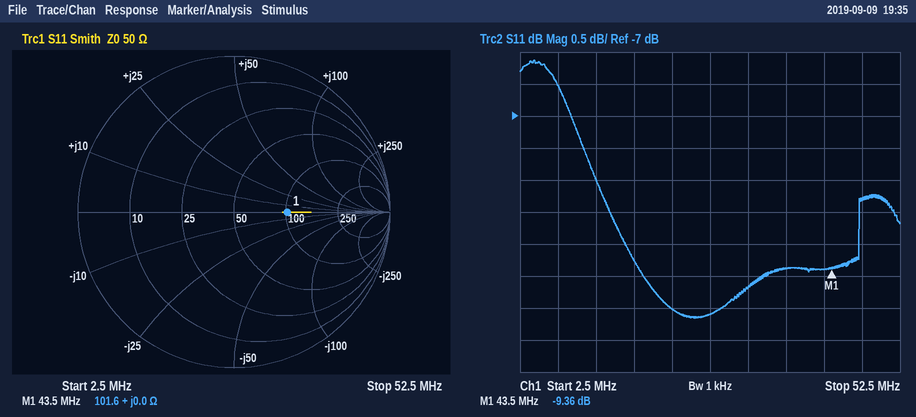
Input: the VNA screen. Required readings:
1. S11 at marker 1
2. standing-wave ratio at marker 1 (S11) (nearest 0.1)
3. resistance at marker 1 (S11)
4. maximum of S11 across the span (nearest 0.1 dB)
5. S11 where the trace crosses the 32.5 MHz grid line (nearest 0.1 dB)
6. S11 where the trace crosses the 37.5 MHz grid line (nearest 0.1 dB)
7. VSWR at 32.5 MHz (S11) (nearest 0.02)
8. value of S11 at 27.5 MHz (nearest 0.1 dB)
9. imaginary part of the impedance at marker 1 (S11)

-9.36 dB
2.0
101.6 Ω
-6.1 dB
-9.7 dB
-9.4 dB
1.98
-10.1 dB
+0.0 Ω
